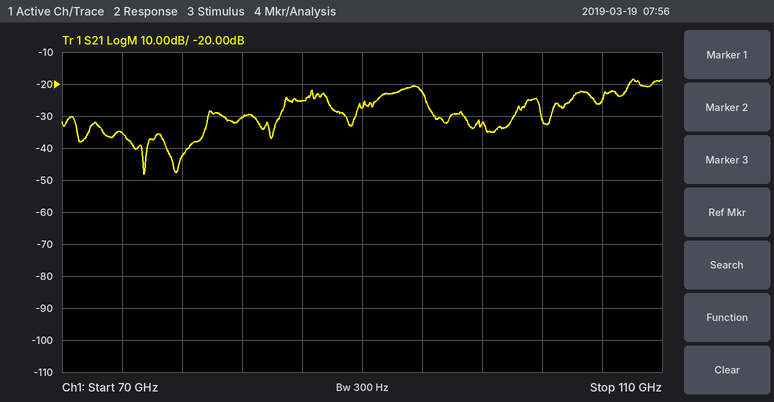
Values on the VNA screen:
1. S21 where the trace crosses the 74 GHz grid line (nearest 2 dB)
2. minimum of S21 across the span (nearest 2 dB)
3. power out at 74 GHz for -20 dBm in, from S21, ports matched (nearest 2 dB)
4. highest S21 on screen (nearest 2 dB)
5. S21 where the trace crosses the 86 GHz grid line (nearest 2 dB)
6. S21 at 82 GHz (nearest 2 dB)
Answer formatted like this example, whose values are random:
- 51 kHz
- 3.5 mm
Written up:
- -36 dB
- -48 dB
- -56 dBm
- -18 dB
- -26 dB
- -30 dB
